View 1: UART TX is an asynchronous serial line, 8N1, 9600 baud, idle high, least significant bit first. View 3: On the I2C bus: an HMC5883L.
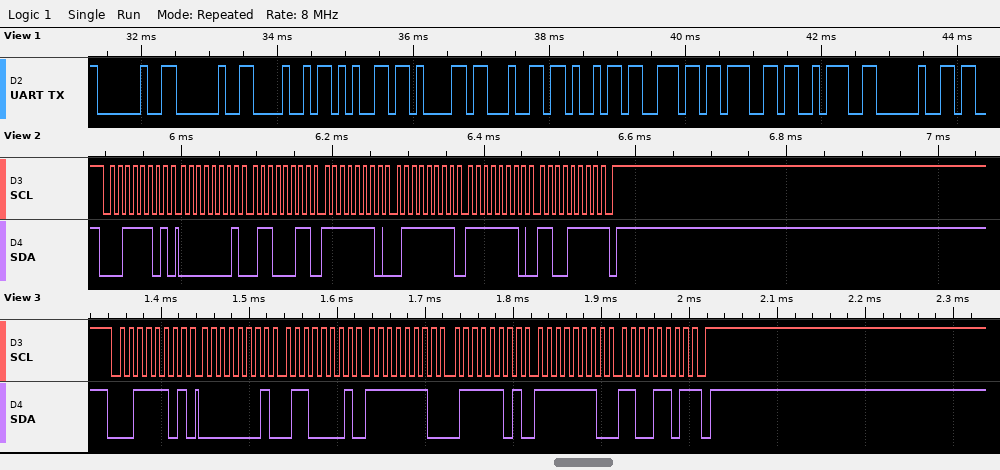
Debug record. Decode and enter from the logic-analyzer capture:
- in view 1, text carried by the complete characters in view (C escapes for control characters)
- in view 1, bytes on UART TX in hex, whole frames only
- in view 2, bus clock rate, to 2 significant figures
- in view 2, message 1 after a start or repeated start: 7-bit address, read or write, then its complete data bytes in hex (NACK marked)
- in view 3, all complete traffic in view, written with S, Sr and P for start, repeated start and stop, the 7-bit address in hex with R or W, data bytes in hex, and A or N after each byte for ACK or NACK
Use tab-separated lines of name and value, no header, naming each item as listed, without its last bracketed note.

in view 1, text carried by the complete characters in view	"  Heading: "
in view 1, bytes on UART TX in hex, whole frames only	20 20 48 65 61 64 69 6E 67 3A 20
in view 2, bus clock rate, to 2 significant figures	100 kHz
in view 2, message 1 after a start or repeated start: 7-bit address, read or write, then its complete data bytes in hex	0x1E read: 01 63 FE 7F FE CF NACK
in view 3, all complete traffic in view, written with S, Sr and P for start, repeated start and stop, the 7-bit address in hex with R or W, data bytes in hex, and A or N after each byte for ACK or NACK	S 1ER A 01 A 61 A FE A 7D A FE A CD N P
